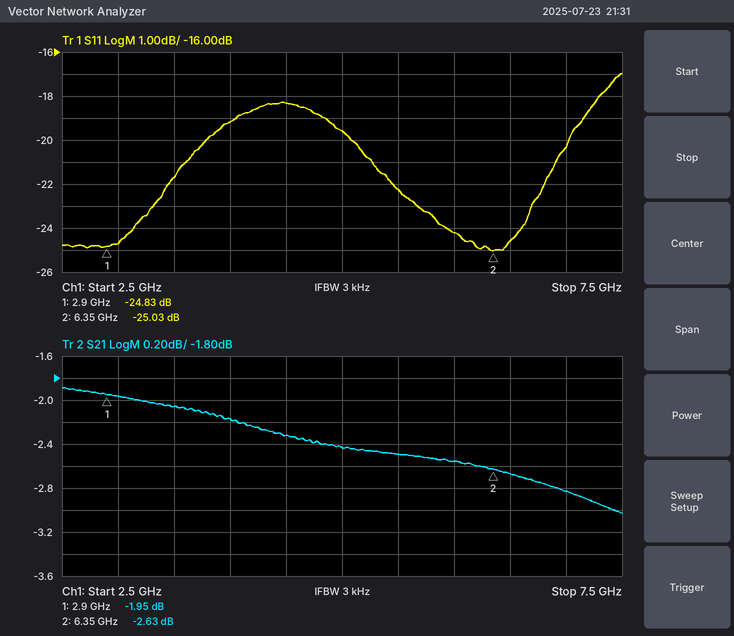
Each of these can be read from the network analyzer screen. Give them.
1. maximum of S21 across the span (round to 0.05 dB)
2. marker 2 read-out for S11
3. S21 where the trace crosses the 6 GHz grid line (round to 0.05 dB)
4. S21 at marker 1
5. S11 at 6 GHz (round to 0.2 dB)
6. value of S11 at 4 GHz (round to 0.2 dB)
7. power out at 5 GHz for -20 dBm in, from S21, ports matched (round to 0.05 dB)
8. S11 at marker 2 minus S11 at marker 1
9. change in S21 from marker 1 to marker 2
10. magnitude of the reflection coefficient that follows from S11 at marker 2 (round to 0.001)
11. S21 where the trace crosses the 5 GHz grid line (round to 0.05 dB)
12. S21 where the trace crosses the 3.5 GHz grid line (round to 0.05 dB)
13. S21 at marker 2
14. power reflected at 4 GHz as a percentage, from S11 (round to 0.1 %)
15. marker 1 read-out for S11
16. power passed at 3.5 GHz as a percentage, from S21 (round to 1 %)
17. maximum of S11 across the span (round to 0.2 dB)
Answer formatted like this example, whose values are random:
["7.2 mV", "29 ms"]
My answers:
["-1.90 dB", "-25.03 dB", "-2.55 dB", "-1.95 dB", "-24.2 dB", "-19.2 dB", "-22.45 dBm", "-0.20 dB", "-0.68 dB", "0.056", "-2.45 dB", "-2.05 dB", "-2.63 dB", "1.2 %", "-24.83 dB", "62 %", "-17.0 dB"]
